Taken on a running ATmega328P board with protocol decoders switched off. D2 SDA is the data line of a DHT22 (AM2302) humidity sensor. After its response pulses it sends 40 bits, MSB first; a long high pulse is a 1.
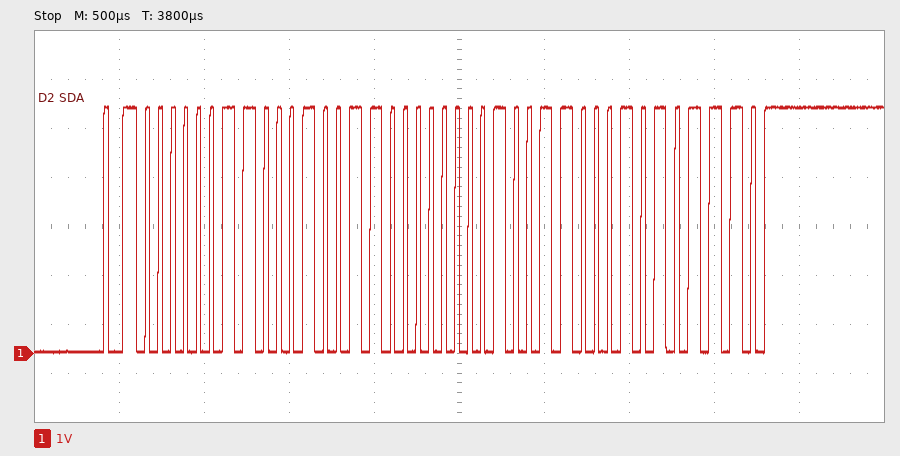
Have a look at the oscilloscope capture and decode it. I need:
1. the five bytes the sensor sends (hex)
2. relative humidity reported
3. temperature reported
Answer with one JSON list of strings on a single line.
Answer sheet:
["03 13 00 98 AE", "78.7 %", "15.2 °C"]
